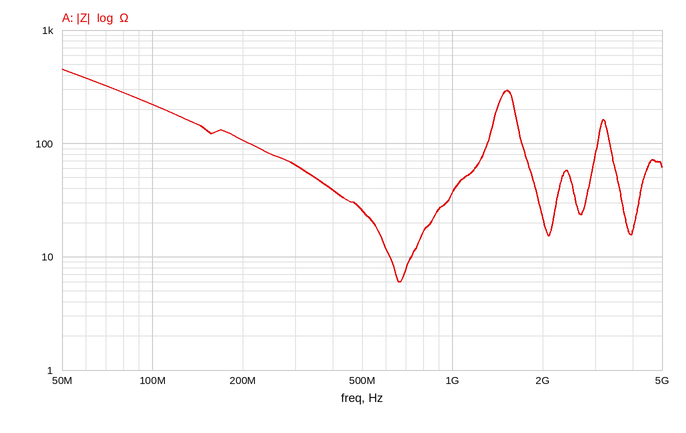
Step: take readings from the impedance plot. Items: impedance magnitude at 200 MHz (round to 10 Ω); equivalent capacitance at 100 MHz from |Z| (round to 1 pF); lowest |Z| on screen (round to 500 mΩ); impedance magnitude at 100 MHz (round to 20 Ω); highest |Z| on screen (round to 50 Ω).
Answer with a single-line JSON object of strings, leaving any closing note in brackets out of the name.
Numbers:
{"impedance magnitude at 200 MHz": "110 Ω", "equivalent capacitance at 100 MHz from |Z|": "7 pF", "lowest |Z| on screen": "6.0 Ω", "impedance magnitude at 100 MHz": "220 Ω", "highest |Z| on screen": "450 Ω"}
